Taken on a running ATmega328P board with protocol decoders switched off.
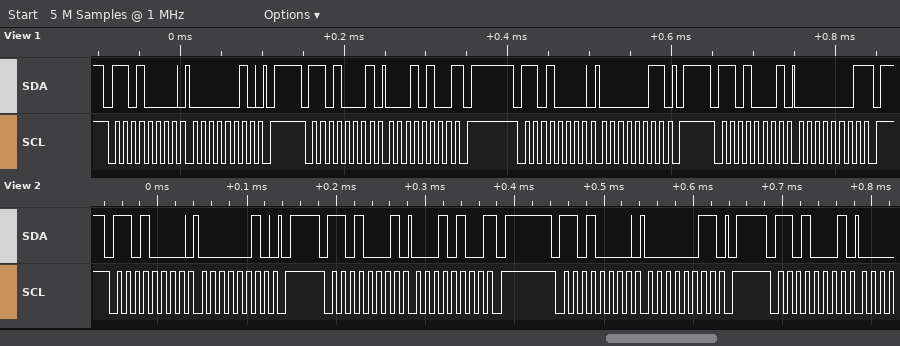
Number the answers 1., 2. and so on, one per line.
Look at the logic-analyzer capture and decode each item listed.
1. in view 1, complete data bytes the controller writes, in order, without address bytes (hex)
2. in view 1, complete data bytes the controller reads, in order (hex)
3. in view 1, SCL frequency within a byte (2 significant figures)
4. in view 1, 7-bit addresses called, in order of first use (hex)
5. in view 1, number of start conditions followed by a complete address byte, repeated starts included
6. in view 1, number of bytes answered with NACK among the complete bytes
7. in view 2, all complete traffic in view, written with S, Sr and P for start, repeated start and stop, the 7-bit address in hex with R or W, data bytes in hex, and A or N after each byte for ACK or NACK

1. 02 03
2. 14 01
3. 100 kHz
4. 0x68
5. 4
6. 2
7. S 68W A 02 A P S 68R A 14 N P S 68W A 03 A P S 68R A
